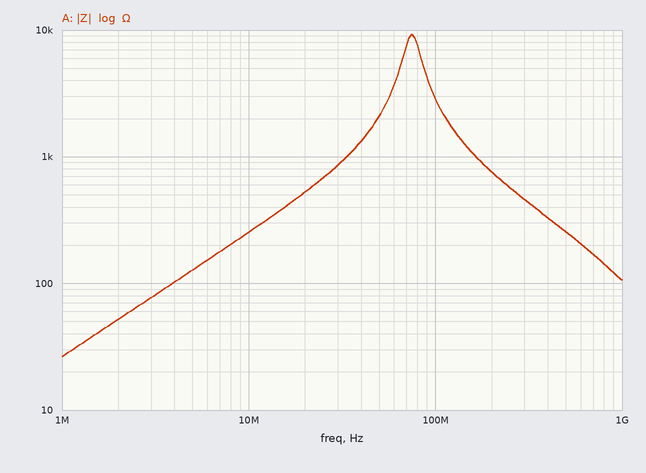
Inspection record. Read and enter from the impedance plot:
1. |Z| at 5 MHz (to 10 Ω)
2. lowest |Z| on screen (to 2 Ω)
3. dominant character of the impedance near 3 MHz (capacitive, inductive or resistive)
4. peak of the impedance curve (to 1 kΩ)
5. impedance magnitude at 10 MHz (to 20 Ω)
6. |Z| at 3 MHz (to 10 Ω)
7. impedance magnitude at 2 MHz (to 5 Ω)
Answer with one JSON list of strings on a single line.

["130 Ω", "26 Ω", "inductive", "9 kΩ", "260 Ω", "80 Ω", "50 Ω"]
